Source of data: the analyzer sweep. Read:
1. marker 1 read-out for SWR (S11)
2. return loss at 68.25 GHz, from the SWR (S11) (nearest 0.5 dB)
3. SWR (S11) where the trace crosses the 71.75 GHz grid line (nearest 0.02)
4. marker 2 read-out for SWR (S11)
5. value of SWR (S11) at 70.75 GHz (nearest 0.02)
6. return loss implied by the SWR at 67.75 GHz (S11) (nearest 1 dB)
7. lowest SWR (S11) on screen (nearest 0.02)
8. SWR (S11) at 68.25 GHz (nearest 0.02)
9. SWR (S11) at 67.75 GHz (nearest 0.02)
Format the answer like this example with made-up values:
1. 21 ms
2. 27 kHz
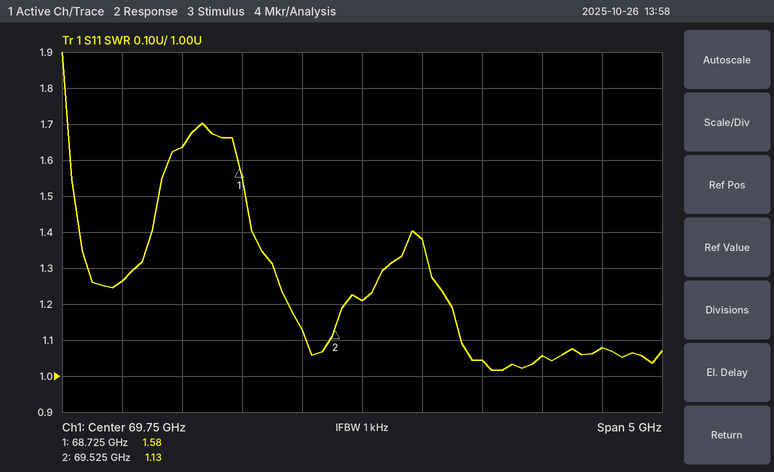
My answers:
1. 1.58
2. 12.5 dB
3. 1.08
4. 1.13
5. 1.04
6. 19 dB
7. 1.02
8. 1.64
9. 1.26
